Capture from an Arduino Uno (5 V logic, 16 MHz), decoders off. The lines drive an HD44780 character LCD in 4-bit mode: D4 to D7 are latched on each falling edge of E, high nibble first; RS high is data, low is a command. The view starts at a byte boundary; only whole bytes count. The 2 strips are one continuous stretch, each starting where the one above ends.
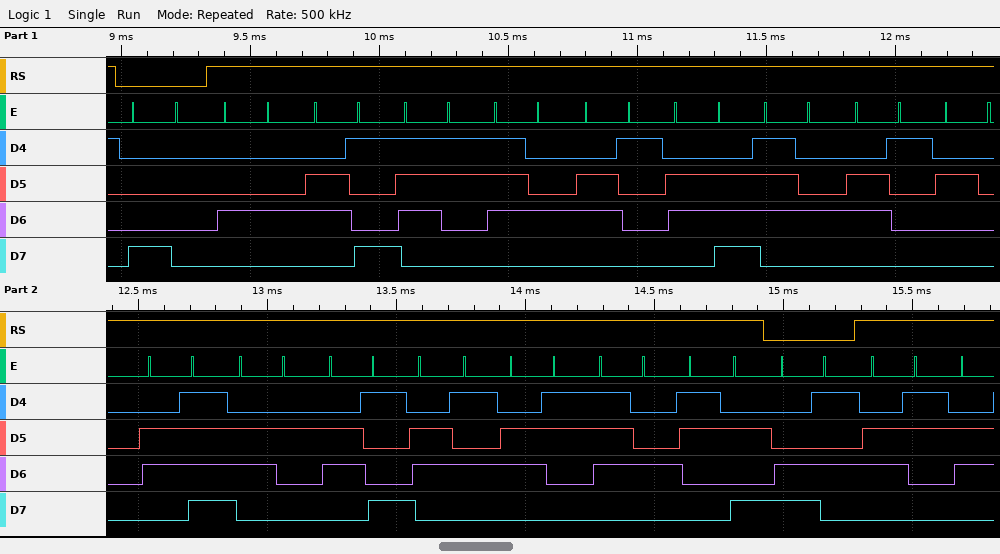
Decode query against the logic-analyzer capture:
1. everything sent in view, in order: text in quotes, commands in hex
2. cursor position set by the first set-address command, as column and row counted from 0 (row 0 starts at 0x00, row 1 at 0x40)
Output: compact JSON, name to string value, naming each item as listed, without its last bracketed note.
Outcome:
{"everything sent in view, in order: text in quotes, commands in hex": "0x80 \"Distanta obiect:\" 0xC5 \"c\"", "cursor position set by the first set-address command, as column and row counted from 0": "column 0, row 0"}
